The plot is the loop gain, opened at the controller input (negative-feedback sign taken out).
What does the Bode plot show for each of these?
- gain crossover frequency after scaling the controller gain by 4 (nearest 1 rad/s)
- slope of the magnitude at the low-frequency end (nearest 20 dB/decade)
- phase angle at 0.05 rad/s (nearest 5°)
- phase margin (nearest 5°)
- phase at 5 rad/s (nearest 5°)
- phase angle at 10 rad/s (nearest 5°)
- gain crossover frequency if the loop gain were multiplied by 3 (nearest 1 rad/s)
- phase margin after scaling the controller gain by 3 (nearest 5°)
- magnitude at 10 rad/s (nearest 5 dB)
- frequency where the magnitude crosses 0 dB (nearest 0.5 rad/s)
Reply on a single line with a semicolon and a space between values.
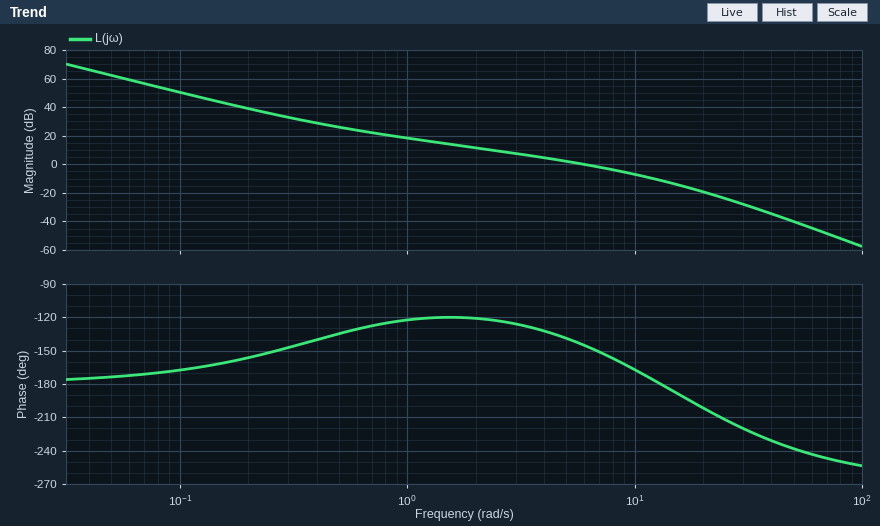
14 rad/s; -40 dB/decade; -175°; 35°; -140°; -165°; 12 rad/s; 5°; -5 dB; 6.0 rad/s
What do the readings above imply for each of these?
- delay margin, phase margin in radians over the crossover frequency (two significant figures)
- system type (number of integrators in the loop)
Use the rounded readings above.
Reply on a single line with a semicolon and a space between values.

0.10 s; 2
